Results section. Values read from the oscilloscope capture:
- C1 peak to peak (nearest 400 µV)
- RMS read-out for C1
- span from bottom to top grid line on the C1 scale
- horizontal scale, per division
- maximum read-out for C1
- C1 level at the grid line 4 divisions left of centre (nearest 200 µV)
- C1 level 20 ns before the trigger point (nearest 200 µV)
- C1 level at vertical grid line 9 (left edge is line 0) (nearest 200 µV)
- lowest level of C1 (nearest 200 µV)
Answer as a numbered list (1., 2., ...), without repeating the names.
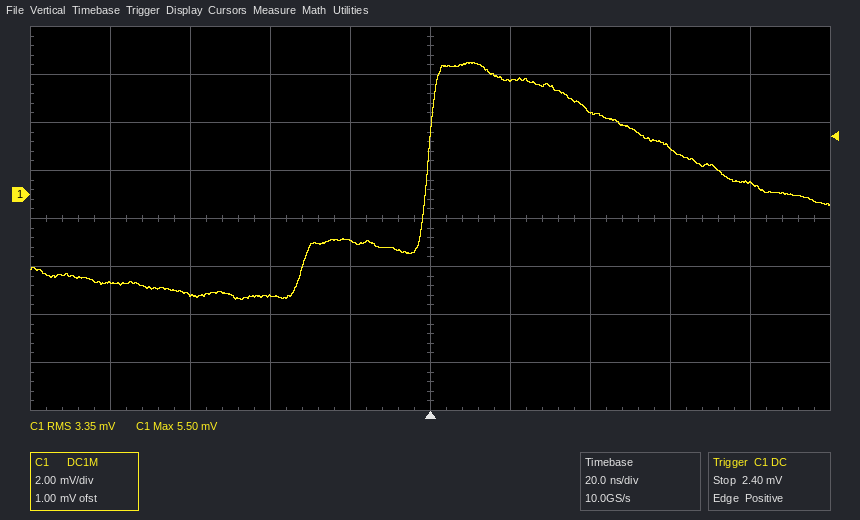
1. 10.0 mV
2. 3.35 mV
3. 16 mV
4. 20 ns
5. 5.50 mV
6. -3.6 mV
7. -2.0 mV
8. 400 µV
9. -4.4 mV
